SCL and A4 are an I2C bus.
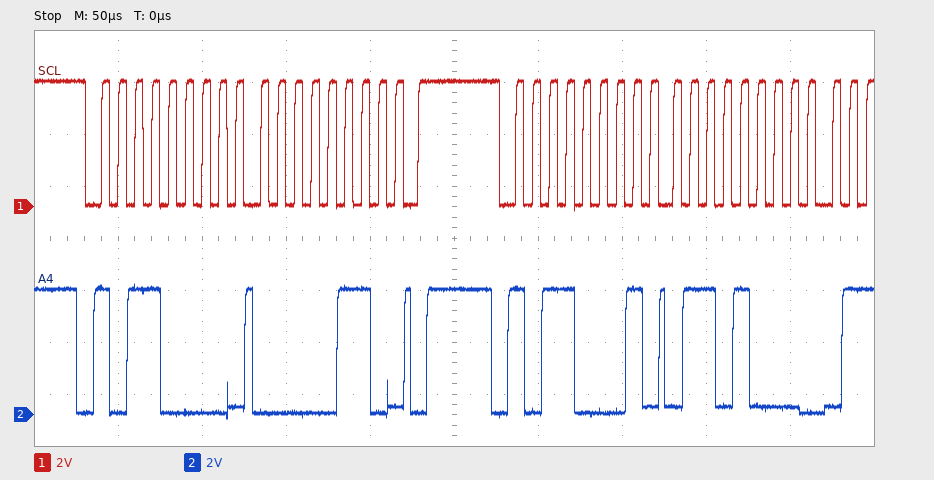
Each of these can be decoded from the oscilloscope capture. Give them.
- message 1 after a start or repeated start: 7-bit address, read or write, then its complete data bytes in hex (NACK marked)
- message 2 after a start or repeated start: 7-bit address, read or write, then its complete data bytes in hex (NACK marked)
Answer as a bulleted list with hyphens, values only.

- 0x58 write: 06
- 0x58 read: 68
